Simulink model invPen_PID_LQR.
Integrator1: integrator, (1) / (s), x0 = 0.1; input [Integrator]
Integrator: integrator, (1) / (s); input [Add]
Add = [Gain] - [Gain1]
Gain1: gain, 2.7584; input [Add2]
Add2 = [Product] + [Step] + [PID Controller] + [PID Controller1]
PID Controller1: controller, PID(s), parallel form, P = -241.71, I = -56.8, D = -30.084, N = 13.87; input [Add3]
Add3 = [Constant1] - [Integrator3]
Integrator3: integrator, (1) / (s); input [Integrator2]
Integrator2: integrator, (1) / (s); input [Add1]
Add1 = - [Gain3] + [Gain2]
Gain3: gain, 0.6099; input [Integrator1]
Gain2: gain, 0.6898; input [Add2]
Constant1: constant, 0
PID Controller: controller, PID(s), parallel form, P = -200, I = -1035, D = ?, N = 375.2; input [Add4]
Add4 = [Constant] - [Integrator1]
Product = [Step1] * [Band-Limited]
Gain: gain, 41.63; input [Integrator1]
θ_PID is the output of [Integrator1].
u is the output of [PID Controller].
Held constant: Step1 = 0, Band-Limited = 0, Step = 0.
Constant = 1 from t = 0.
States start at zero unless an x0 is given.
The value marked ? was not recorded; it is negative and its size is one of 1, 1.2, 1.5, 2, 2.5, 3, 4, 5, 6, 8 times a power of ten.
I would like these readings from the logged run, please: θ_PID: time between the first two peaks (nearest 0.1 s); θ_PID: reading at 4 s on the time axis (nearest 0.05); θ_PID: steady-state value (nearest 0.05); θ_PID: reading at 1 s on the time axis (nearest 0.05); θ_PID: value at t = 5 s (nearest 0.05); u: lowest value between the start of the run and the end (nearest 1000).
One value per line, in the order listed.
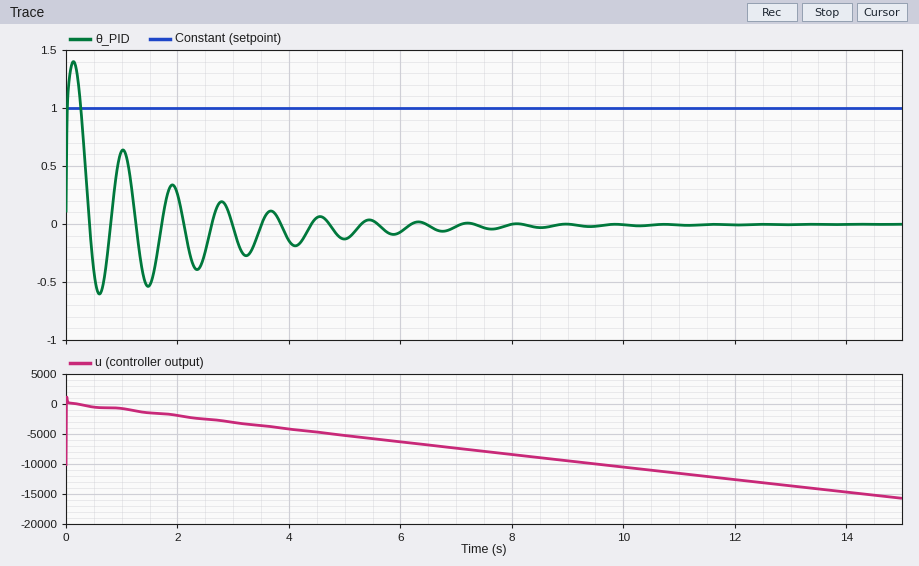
0.9 s
-0.15
0.00
0.65
-0.15
-16000
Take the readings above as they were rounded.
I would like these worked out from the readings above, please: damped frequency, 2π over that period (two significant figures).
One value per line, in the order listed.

7.0 rad/s
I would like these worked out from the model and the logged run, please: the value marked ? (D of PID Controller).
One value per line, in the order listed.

-30
